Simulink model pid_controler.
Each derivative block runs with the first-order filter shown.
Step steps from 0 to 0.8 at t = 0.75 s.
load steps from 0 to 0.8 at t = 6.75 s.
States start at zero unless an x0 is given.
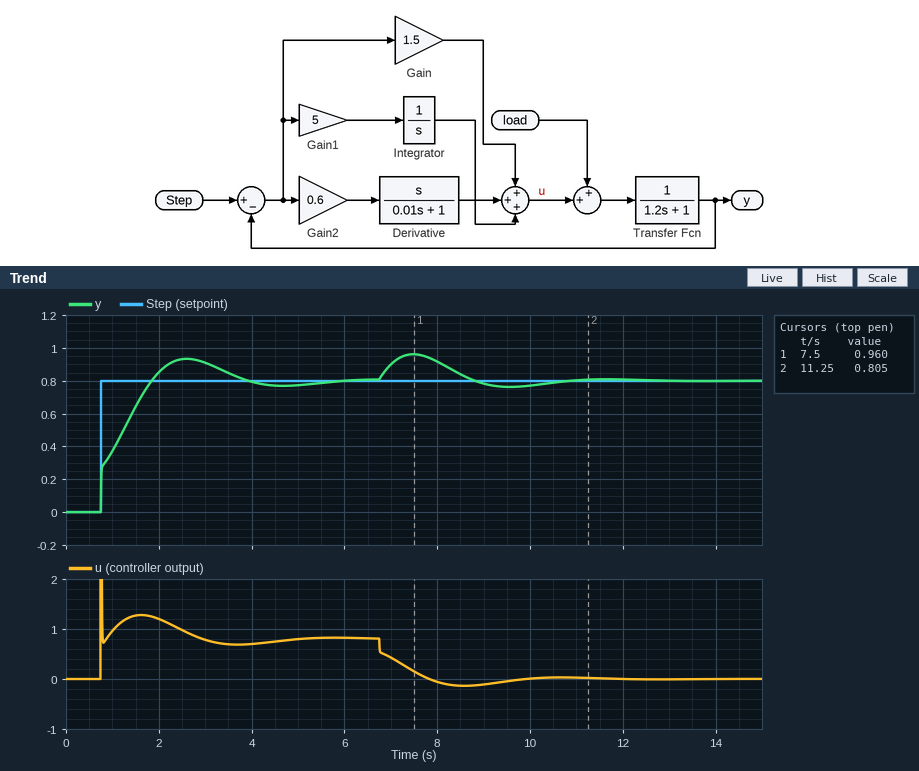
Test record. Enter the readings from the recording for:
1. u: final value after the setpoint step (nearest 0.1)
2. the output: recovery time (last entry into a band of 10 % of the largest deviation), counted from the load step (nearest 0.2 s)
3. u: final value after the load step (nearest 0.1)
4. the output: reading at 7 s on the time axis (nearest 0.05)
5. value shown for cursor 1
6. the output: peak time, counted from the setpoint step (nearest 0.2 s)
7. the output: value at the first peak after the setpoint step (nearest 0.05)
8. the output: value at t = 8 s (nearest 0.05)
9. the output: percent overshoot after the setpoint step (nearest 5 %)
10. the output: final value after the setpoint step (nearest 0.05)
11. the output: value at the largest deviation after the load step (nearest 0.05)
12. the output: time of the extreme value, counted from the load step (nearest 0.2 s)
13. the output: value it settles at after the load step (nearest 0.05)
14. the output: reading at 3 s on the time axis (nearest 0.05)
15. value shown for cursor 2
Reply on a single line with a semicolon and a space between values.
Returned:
0.8; 3.6 s; 0.0; 0.90; 0.960; 1.8 s; 0.95; 0.90; 15 %; 0.80; 0.95; 0.8 s; 0.80; 0.90; 0.805
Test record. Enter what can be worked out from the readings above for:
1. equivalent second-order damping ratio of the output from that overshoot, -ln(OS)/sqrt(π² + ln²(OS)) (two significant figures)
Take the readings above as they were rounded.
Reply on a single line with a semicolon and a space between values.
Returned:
0.52
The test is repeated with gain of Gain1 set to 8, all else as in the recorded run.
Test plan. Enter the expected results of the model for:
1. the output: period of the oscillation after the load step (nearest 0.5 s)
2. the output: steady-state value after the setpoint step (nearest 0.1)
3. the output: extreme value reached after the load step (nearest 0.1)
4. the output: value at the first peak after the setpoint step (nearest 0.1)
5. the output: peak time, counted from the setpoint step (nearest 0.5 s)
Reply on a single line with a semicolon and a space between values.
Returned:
3.0 s; 0.8; 0.9; 1.0; 1.5 s
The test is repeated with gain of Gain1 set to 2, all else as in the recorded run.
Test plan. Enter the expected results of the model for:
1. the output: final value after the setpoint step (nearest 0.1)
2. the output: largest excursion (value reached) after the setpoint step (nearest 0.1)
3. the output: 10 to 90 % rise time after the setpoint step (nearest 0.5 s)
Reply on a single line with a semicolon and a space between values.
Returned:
0.8; 0.8; 1.5 s
